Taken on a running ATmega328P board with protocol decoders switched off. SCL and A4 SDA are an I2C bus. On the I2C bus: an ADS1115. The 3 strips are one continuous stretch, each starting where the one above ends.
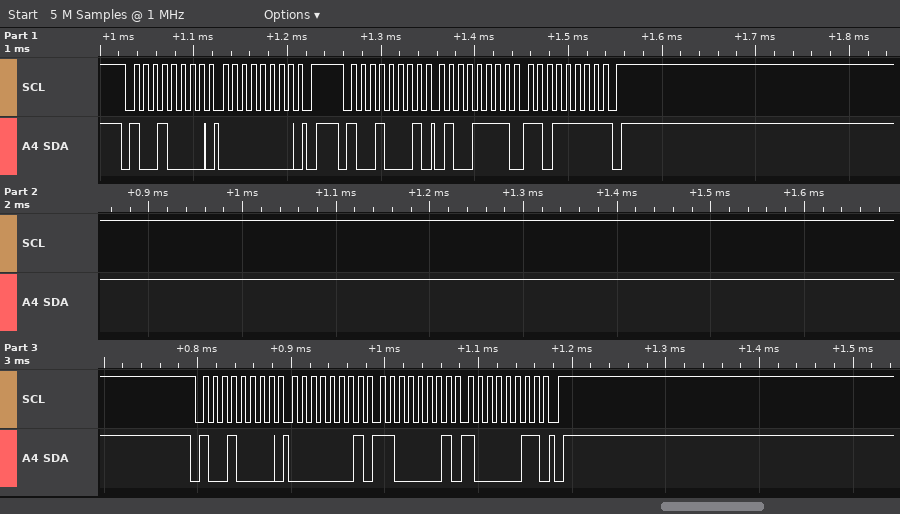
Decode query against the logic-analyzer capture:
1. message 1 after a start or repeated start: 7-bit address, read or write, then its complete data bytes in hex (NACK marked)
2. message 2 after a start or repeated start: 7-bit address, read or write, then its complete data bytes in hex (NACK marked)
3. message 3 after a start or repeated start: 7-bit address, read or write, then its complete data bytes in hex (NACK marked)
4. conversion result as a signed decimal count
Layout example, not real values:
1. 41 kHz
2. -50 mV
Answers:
1. 0x48 write: 00
2. 0x48 read: 4F DF NACK
3. 0x48 write: 01 C1 83
4. 20447
